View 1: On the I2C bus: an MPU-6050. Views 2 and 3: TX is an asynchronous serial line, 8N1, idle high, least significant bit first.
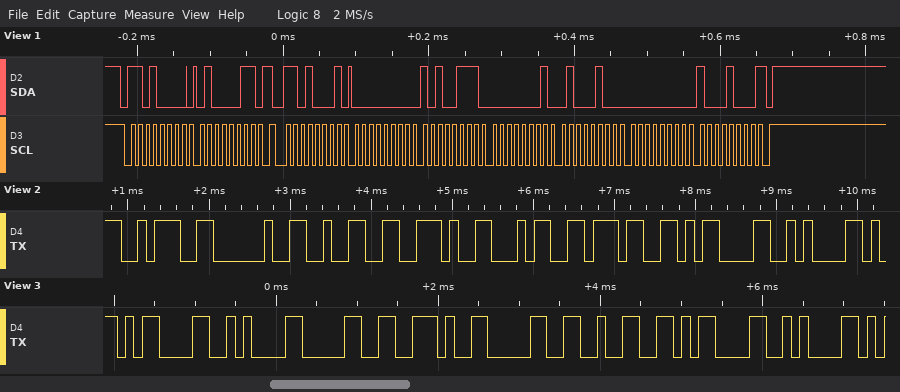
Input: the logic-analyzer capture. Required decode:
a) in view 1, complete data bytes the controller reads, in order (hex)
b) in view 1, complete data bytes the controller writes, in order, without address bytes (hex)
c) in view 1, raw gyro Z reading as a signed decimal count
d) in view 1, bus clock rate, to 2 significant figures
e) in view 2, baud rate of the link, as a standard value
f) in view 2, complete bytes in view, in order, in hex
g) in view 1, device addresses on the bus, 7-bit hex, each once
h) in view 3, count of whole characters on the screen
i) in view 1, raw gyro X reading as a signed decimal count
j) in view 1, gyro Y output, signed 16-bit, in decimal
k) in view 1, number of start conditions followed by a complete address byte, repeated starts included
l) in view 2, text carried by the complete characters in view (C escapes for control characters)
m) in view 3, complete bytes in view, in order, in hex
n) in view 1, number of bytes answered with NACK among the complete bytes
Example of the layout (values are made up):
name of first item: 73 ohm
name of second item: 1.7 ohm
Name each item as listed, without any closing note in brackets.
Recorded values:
in view 1, complete data bytes the controller reads, in order: 00 A7 01 44 00 88
in view 1, complete data bytes the controller writes, in order, without address bytes: 43
in view 1, raw gyro Z reading as a signed decimal count: 136
in view 1, bus clock rate, to 2 significant figures: 100 kHz
in view 2, baud rate of the link, as a standard value: 9600 baud
in view 2, complete bytes in view, in order, in hex: 3A 20 32 2E 34 37 0D 0A
in view 1, device addresses on the bus, 7-bit hex, each once: 0x68
in view 3, count of whole characters on the screen: 8
in view 1, raw gyro X reading as a signed decimal count: 167
in view 1, gyro Y output, signed 16-bit, in decimal: 324
in view 1, number of start conditions followed by a complete address byte, repeated starts included: 2
in view 2, text carried by the complete characters in view: ": 2.47\r\n"
in view 3, complete bytes in view, in order, in hex: 0D 0A 30 2E 30 32 0D 0A
in view 1, number of bytes answered with NACK among the complete bytes: 1
